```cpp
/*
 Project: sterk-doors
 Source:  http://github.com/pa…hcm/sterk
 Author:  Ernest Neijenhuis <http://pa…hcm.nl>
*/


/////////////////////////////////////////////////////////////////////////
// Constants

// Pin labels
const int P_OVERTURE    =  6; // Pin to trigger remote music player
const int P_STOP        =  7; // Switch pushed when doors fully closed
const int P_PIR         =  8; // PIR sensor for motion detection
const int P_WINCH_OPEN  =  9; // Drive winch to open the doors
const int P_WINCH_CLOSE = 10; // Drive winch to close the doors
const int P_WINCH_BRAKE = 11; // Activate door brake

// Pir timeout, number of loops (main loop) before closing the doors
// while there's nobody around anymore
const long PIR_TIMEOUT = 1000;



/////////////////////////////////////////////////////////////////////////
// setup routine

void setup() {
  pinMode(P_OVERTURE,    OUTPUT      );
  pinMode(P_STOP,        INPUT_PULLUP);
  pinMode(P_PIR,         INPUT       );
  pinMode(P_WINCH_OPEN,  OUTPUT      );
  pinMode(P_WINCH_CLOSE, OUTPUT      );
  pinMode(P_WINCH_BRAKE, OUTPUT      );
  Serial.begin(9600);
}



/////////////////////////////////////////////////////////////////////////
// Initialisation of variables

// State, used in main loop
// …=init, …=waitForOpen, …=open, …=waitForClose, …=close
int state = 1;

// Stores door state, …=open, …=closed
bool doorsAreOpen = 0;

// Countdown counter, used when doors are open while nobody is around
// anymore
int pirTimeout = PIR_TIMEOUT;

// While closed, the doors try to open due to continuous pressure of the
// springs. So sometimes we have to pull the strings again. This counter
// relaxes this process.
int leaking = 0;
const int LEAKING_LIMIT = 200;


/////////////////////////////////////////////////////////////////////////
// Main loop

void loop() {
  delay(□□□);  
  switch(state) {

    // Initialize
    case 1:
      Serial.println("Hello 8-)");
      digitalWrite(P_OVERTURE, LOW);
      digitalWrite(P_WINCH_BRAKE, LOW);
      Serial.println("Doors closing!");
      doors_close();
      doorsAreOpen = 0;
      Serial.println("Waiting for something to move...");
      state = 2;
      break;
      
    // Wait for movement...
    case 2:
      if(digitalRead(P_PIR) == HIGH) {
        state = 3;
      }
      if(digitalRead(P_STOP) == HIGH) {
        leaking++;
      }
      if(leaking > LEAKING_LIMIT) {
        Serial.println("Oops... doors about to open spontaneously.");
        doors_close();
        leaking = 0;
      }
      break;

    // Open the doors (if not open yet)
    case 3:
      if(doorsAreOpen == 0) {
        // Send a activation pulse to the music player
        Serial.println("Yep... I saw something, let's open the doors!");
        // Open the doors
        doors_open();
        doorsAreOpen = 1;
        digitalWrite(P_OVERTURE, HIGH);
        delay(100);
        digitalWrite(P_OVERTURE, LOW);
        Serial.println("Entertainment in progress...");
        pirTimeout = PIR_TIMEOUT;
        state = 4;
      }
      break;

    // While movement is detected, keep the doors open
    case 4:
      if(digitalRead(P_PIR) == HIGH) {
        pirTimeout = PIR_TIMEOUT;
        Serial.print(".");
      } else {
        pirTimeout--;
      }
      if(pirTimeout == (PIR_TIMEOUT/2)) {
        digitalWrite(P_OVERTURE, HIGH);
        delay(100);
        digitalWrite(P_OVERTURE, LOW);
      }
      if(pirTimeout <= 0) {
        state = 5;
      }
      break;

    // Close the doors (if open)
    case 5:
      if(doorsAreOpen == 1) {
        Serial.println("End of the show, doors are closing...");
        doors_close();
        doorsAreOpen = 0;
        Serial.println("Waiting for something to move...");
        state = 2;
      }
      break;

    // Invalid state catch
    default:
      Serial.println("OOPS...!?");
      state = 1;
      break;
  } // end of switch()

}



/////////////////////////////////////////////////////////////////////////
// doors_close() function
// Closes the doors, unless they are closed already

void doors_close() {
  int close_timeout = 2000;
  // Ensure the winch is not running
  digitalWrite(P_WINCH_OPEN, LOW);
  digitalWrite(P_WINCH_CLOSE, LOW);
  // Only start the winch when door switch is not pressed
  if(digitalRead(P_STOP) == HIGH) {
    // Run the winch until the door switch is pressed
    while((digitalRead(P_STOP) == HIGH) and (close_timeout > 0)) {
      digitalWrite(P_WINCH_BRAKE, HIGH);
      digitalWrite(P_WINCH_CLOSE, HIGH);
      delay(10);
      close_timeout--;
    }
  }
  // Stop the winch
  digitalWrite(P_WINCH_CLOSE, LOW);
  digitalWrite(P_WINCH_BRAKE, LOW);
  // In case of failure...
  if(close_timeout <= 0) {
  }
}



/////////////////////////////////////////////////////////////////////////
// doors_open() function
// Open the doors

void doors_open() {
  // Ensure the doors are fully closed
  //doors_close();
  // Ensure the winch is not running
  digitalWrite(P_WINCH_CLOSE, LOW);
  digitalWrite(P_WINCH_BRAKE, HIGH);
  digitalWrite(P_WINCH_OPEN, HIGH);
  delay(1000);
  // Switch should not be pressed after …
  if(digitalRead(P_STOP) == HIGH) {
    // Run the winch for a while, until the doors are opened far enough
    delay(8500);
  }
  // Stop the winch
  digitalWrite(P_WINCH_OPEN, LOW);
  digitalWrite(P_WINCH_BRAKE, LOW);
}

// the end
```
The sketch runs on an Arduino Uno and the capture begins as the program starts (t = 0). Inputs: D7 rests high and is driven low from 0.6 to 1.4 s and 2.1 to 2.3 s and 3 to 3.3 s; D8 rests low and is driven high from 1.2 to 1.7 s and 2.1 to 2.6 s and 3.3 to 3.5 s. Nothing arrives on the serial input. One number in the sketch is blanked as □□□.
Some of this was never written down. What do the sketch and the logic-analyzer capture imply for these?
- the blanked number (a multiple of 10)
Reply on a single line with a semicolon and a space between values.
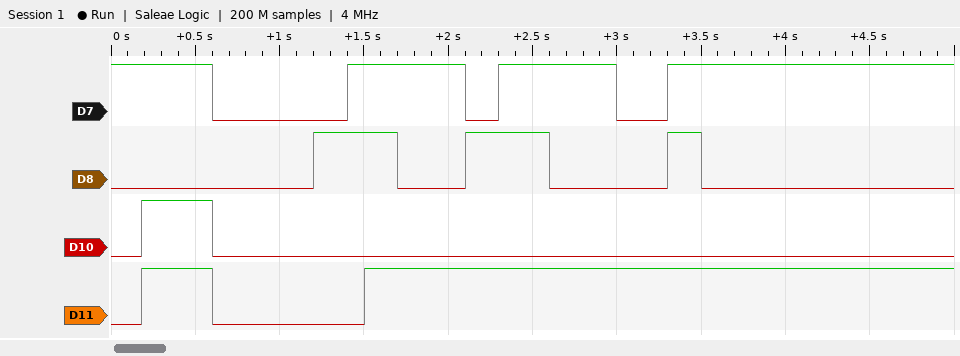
180
